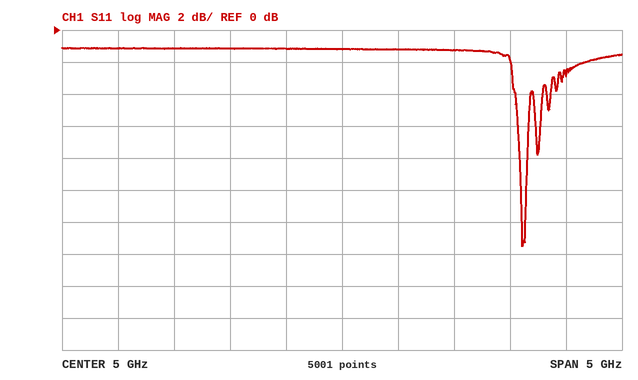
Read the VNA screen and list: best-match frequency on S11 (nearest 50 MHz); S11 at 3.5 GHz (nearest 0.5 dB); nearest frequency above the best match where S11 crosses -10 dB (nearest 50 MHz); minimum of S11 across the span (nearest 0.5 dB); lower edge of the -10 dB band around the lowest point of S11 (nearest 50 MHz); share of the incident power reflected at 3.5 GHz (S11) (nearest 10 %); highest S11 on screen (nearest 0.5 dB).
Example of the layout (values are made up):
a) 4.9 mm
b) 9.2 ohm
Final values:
a) 6.60 GHz
b) -1.0 dB
c) 6.65 GHz
d) -13.5 dB
e) 6.60 GHz
f) 80 %
g) -1.0 dB
